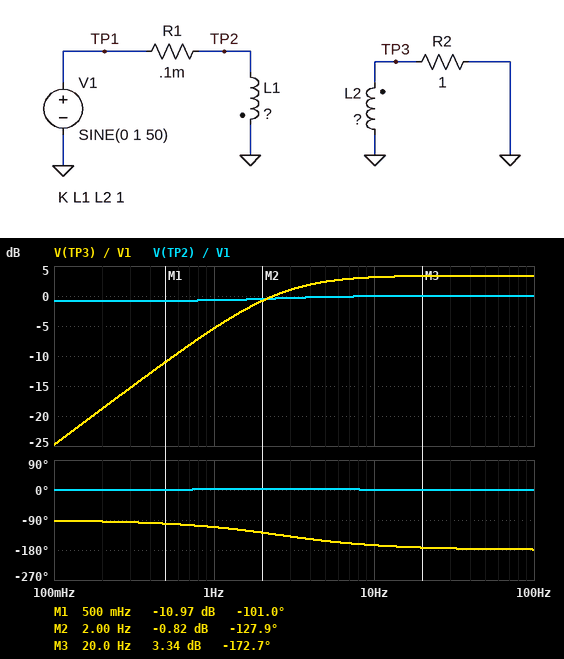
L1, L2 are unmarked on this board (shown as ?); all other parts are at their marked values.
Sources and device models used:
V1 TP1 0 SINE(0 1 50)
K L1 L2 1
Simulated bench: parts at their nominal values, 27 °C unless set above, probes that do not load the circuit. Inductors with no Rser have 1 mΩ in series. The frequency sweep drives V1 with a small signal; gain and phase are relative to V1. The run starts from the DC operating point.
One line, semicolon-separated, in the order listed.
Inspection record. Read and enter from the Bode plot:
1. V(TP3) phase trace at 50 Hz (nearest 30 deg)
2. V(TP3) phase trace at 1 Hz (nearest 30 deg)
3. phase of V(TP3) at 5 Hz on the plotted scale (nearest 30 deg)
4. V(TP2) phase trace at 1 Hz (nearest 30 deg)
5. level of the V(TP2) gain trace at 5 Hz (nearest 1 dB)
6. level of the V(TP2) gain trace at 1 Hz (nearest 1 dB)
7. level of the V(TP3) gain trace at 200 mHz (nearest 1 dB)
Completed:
-180 deg; -120 deg; -150 deg; 0 deg; 0 dB; -1 dB; -19 dB
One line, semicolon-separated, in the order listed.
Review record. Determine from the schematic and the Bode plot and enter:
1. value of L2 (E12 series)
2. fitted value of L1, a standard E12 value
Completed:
150 µH; 68 µH
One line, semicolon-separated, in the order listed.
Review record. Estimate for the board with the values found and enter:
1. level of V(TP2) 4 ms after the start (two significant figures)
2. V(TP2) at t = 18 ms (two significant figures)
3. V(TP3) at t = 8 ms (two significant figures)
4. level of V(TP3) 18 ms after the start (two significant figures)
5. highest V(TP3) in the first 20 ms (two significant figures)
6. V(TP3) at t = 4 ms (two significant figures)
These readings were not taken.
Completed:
950 mV; -590 mV; -740 mV; 860 mV; 1.5 V; -1.4 V
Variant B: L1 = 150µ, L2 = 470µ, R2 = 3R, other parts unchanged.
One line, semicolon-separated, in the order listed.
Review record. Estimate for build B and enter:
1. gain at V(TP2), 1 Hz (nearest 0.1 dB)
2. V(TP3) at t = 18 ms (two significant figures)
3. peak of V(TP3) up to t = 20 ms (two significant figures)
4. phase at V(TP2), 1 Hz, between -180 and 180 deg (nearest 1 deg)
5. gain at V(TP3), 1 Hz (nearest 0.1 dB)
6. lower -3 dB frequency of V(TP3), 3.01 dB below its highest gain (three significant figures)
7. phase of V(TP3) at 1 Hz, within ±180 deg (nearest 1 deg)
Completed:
-0.5 dB; 1.0 V; 1.8 V; 3 deg; 1.2 dB; 1.17 Hz; -131 deg
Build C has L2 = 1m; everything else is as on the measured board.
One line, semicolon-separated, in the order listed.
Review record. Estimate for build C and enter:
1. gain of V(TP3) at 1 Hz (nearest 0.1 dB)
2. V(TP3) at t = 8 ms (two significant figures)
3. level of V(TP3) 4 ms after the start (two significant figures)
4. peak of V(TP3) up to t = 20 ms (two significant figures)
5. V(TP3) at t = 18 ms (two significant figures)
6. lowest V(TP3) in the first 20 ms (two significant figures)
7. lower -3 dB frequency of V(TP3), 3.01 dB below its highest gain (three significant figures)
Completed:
2.8 dB; -1.9 V; -3.5 V; 3.9 V; 2.2 V; -3.6 V; 2.53 Hz
